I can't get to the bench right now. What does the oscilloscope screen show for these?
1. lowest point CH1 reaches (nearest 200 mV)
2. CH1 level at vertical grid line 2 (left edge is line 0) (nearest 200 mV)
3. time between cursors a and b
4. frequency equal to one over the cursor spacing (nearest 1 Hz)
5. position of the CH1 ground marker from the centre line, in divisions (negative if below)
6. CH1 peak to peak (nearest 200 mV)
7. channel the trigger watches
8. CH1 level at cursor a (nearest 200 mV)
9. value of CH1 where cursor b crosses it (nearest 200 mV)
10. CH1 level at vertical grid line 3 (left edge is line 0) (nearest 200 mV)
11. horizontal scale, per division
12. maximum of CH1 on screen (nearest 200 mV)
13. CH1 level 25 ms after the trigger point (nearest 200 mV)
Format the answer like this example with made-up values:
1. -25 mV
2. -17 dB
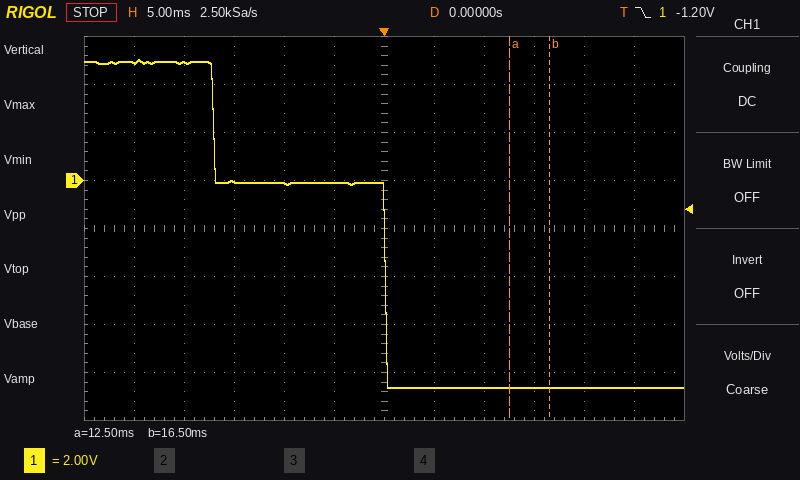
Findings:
1. -8.6 V
2. 5.0 V
3. 4.0 ms
4. 250 Hz
5. +1.0 div
6. 13.6 V
7. CH1
8. -8.6 V
9. -8.6 V
10. 0.0 V
11. 5 ms
12. 5.0 V
13. -8.6 V
